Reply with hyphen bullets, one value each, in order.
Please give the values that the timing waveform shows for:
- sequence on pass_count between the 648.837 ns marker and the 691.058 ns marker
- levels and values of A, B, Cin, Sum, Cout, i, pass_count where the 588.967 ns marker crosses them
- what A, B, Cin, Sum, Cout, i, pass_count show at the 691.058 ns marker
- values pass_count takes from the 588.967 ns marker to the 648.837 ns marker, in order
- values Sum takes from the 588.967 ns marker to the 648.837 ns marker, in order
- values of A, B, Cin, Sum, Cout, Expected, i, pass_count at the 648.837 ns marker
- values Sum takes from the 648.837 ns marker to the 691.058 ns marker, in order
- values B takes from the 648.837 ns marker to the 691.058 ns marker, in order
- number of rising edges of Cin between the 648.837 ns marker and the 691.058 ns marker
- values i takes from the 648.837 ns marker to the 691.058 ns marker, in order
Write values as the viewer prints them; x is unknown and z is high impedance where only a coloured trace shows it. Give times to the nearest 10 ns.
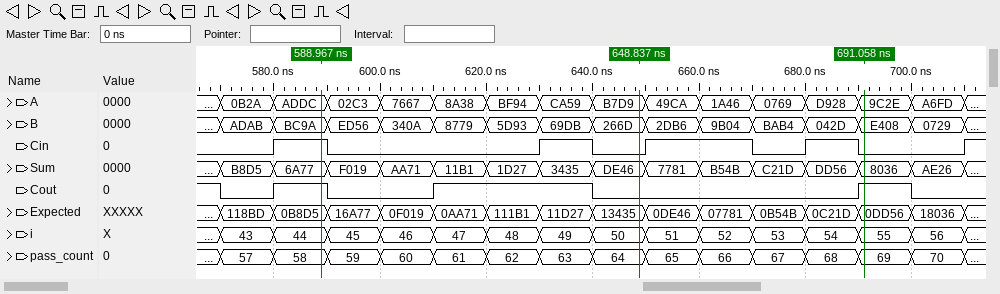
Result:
- 64, 65, 66, 67, 68, 69
- A=ADDC, B=BC9A, Cin=1, Sum=6A77, Cout=1, i=44, pass_count=58
- A=9C2E, B=E408, Cin=0, Sum=8036, Cout=1, i=55, pass_count=69
- 58, 59, 60, 61, 62, 63, 64
- 6A77, F019, AA71, 11B1, 1D27, 3435, DE46
- A=B7D9, B=266D, Cin=0, Sum=DE46, Cout=0, Expected=13435, i=50, pass_count=64
- DE46, 7781, B54B, C21D, DD56, 8036
- 266D, 2DB6, 9B04, BAB4, 042D, E408
- 2
- 50, 51, 52, 53, 54, 55
